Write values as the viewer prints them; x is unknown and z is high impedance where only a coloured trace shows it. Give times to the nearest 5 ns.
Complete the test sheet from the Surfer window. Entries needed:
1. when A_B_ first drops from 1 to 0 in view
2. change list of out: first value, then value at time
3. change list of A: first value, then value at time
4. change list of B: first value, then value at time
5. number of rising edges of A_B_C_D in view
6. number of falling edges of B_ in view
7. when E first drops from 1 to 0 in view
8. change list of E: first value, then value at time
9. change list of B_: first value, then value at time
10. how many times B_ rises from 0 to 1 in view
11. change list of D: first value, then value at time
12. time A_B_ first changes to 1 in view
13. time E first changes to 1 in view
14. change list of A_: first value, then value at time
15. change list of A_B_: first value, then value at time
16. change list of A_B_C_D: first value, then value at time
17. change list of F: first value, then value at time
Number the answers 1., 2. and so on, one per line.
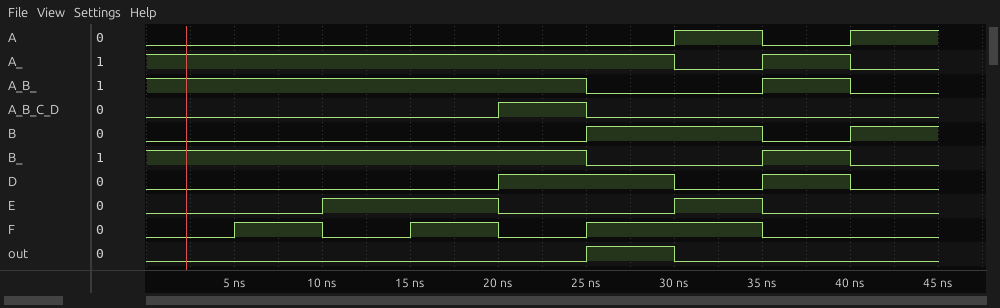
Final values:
1. 25 ns
2. 0, 1 at 25 ns, 0 at 30 ns
3. 0, 1 at 30 ns, 0 at 35 ns, 1 at 40 ns
4. 0, 1 at 25 ns, 0 at 35 ns, 1 at 40 ns
5. 1
6. 2
7. 20 ns
8. 0, 1 at 10 ns, 0 at 20 ns, 1 at 30 ns, 0 at 35 ns
9. 1, 0 at 25 ns, 1 at 35 ns, 0 at 40 ns
10. 1
11. 0, 1 at 20 ns, 0 at 30 ns, 1 at 35 ns, 0 at 40 ns
12. 35 ns
13. 10 ns
14. 1, 0 at 30 ns, 1 at 35 ns, 0 at 40 ns
15. 1, 0 at 25 ns, 1 at 35 ns, 0 at 40 ns
16. 0, 1 at 20 ns, 0 at 25 ns
17. 0, 1 at 5 ns, 0 at 10 ns, 1 at 15 ns, 0 at 20 ns, 1 at 25 ns, 0 at 35 ns
